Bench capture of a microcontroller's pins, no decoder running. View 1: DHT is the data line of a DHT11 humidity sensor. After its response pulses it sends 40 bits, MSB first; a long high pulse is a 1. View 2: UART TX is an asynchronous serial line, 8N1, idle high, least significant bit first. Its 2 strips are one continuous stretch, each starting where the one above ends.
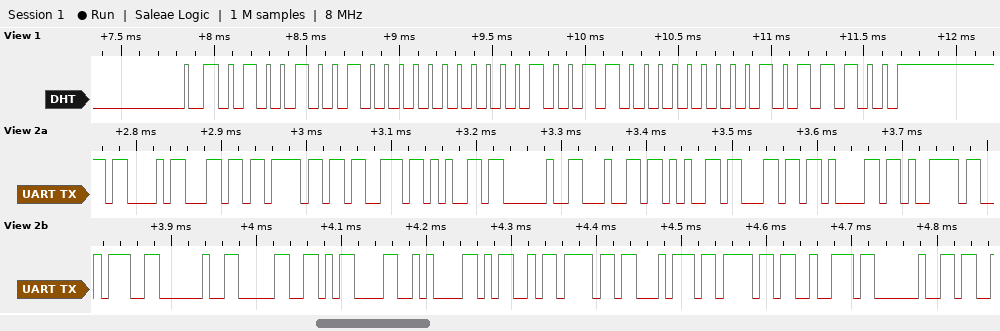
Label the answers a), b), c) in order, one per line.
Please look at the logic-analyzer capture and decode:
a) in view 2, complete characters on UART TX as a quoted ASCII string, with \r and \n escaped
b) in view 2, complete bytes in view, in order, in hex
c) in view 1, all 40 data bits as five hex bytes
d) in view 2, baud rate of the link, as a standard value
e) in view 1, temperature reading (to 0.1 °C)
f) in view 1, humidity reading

a) "Close delay: 0\r\nMotor "
b) 43 6C 6F 73 65 20 64 65 6C 61 79 3A 20 30 0D 0A 4D 6F 74 6F 72 20
c) 49 00 13 00 5C
d) 115200 baud
e) 19.0 °C
f) 73 %
